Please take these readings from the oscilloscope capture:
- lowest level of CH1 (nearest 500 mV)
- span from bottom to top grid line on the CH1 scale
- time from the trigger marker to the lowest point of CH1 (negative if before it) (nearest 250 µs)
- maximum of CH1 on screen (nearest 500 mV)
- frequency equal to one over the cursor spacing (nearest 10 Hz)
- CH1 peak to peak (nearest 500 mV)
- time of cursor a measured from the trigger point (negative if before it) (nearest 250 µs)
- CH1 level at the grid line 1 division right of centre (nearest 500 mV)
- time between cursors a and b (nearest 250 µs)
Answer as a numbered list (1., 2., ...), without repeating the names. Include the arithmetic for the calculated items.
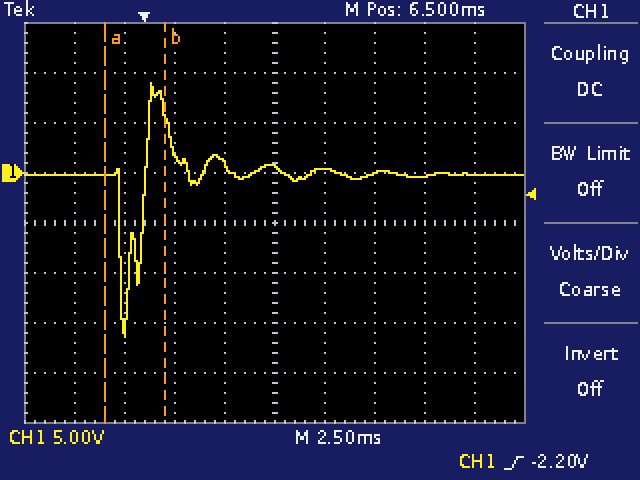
1. -16.5 V
2. 40 V
3. -1.00 ms
4. 9.0 V
5. 1 / 3.00 ms ≈ 330 Hz
6. 9.0 V − (-16.5 V) = 25.5 V
7. -2.00 ms
8. 500 mV
9. 3.00 ms
